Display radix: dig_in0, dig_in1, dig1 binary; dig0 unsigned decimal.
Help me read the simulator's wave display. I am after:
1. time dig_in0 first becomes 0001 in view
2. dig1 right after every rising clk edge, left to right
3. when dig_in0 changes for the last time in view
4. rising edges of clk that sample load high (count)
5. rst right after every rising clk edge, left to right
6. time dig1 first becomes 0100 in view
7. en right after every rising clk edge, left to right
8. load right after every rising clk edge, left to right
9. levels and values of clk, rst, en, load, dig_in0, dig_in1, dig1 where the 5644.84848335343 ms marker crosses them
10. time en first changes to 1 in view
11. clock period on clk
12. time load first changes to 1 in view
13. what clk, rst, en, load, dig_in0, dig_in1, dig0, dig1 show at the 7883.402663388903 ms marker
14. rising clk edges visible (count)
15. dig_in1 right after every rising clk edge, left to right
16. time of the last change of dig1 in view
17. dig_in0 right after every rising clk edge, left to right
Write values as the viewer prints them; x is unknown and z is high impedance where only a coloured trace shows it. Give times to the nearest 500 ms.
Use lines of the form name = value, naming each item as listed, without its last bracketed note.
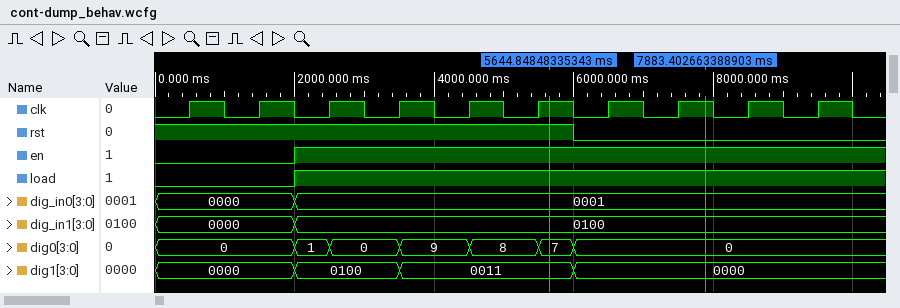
time dig_in0 first becomes 0001 in view = 2000 ms
dig1 right after every rising clk edge, left to right = 0000, 0000, 0100, 0011, 0011, 0011, 0000, 0000, 0000, 0000
when dig_in0 changes for the last time in view = 2000 ms
rising edges of clk that sample load high = 8
rst right after every rising clk edge, left to right = 1 1 1 1 1 1 0 0 0 0
time dig1 first becomes 0100 in view = 2000 ms
en right after every rising clk edge, left to right = 0 0 1 1 1 1 1 1 1 1
load right after every rising clk edge, left to right = 0 0 1 1 1 1 1 1 1 1
levels and values of clk, rst, en, load, dig_in0, dig_in1, dig1 where the 5644.84848335343 ms marker crosses them = clk=1, rst=1, en=1, load=1, dig_in0=0001, dig_in1=0100, dig1=0011
time en first changes to 1 in view = 2000 ms
clock period on clk = 1000 ms
time load first changes to 1 in view = 2000 ms
what clk, rst, en, load, dig_in0, dig_in1, dig0, dig1 show at the 7883.402663388903 ms marker = clk=1, rst=0, en=1, load=1, dig_in0=0001, dig_in1=0100, dig0=0, dig1=0000
rising clk edges visible = 10
dig_in1 right after every rising clk edge, left to right = 0000, 0000, 0100, 0100, 0100, 0100, 0100, 0100, 0100, 0100
time of the last change of dig1 in view = 6000 ms
dig_in0 right after every rising clk edge, left to right = 0000, 0000, 0001, 0001, 0001, 0001, 0001, 0001, 0001, 0001
